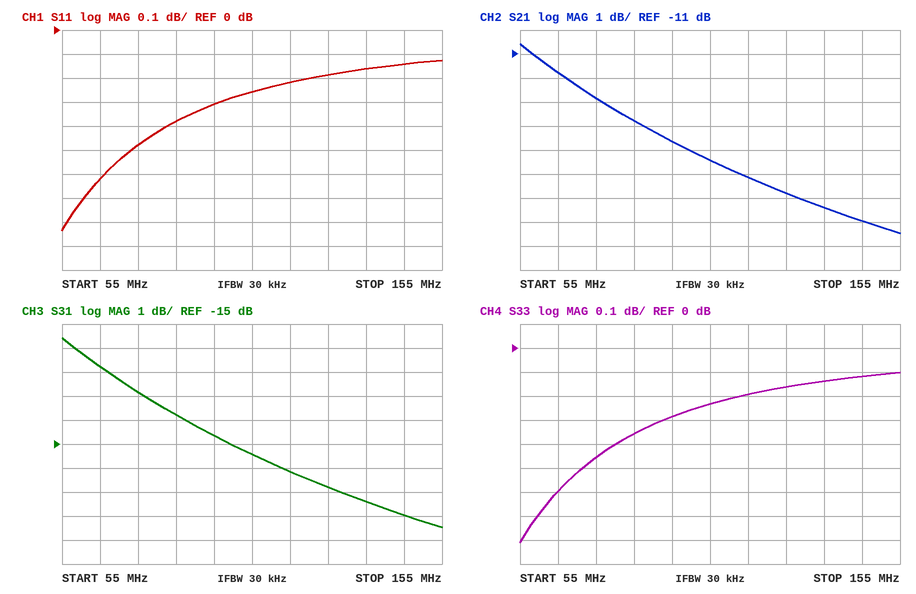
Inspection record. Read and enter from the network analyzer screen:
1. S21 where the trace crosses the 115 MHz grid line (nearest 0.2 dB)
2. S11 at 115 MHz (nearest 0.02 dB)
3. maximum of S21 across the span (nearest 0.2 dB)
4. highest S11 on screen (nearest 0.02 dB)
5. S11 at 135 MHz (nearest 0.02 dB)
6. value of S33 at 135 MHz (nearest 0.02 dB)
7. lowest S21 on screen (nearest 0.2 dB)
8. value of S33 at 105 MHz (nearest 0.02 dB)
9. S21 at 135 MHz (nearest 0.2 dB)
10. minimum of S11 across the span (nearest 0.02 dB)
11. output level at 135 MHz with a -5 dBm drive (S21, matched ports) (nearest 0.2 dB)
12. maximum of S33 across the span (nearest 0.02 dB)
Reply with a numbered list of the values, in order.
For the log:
1. -16.2 dB
2. -0.22 dB
3. -10.6 dB
4. -0.12 dB
5. -0.16 dB
6. -0.14 dB
7. -18.4 dB
8. -0.24 dB
9. -17.4 dB
10. -0.84 dB
11. -22.4 dBm
12. -0.10 dB
